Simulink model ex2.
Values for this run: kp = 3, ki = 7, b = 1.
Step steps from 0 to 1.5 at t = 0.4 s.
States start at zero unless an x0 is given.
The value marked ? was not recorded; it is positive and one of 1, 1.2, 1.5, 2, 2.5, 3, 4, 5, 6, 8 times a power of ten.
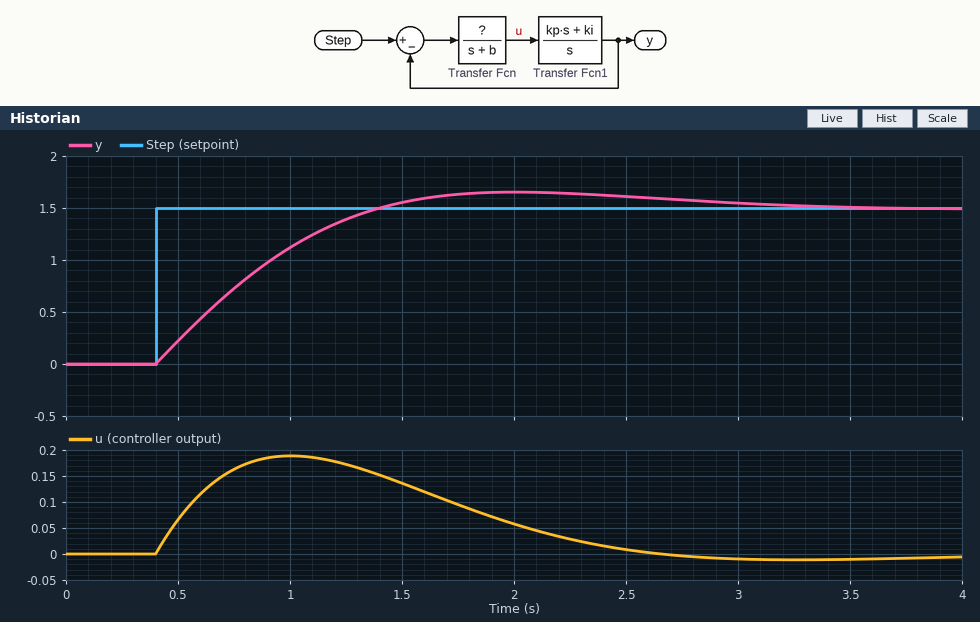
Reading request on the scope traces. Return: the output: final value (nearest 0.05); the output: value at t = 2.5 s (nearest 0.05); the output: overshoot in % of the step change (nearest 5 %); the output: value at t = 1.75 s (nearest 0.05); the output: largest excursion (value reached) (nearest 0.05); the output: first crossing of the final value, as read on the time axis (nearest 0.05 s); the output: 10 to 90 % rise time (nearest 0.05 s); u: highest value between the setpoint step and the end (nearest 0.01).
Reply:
1.50
1.60
10 %
1.65
1.65
1.40 s
0.75 s
0.19
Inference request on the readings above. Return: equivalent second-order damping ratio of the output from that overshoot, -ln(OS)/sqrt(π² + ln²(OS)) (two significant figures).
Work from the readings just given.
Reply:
0.59
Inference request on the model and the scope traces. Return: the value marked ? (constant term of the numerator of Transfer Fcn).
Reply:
0.5
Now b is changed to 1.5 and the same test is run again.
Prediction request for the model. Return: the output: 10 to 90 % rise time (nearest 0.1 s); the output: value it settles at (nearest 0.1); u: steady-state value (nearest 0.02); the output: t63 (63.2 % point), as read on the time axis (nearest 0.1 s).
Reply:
0.9 s
1.5
0.00
0.9 s
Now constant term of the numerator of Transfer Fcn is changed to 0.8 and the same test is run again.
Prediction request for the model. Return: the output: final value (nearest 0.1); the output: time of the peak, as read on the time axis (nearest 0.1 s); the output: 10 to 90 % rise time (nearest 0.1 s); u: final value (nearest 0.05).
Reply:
1.5
1.6 s
0.5 s
0.00
